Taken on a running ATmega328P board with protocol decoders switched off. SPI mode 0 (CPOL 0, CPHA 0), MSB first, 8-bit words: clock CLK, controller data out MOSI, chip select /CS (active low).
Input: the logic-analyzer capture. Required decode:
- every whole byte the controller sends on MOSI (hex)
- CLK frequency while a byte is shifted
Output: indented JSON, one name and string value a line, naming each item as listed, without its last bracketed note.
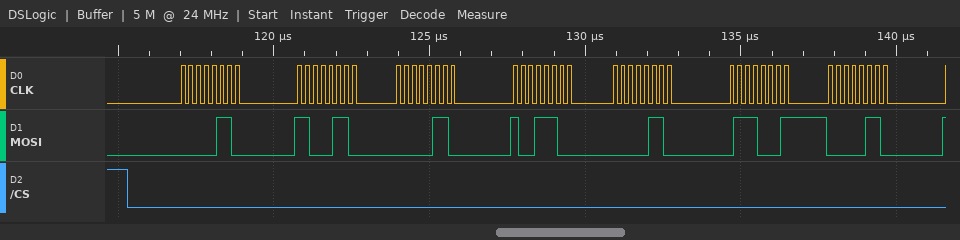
{
  "every whole byte the controller sends on MOSI": "06 C6 06 9C 06 71 06",
  "CLK frequency while a byte is shifted": "4 MHz"
}
